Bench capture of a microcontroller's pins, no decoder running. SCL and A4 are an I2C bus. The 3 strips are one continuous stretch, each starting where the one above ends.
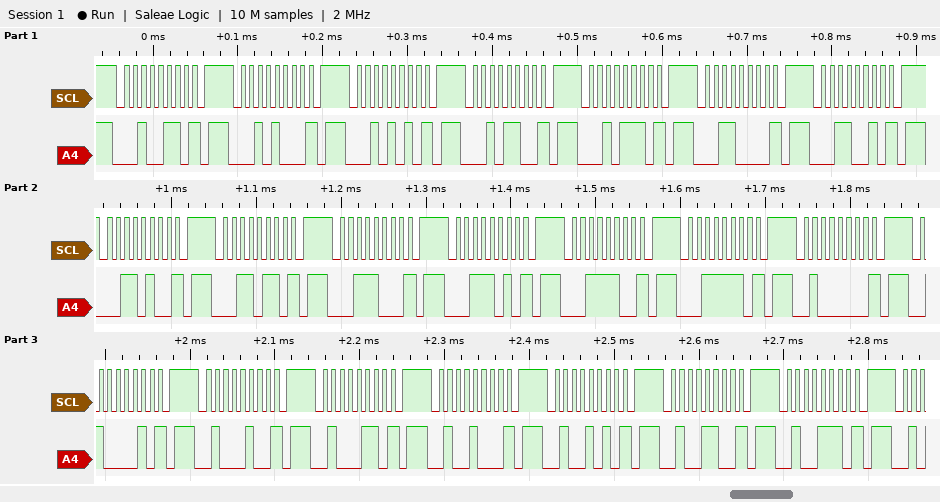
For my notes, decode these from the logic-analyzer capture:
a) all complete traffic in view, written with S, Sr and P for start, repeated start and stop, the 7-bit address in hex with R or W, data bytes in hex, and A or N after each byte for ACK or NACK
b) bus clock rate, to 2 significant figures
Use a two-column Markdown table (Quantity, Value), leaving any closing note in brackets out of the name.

| Quantity | Value |
|---|---|
| all complete traffic in view, written with S, Sr and P for start, repeated start and stop, the 7-bit address in hex with R or W, data bytes in hex, and A or N after each byte for ACK or NACK | S 13W N P S 14W N P S 15W N P S 16W N P S 17W N P S 18W N P S 19W N P S 1AW N P S 1BW N P S 1CW N P S 1DW N P S 1EW N P S 1FW N P S 20W N P S 21W N P S 22W N P S 23W N P S 24W N P S 25W N P S 26W N P S 27W N P |
| bus clock rate, to 2 significant figures | 100 kHz |
